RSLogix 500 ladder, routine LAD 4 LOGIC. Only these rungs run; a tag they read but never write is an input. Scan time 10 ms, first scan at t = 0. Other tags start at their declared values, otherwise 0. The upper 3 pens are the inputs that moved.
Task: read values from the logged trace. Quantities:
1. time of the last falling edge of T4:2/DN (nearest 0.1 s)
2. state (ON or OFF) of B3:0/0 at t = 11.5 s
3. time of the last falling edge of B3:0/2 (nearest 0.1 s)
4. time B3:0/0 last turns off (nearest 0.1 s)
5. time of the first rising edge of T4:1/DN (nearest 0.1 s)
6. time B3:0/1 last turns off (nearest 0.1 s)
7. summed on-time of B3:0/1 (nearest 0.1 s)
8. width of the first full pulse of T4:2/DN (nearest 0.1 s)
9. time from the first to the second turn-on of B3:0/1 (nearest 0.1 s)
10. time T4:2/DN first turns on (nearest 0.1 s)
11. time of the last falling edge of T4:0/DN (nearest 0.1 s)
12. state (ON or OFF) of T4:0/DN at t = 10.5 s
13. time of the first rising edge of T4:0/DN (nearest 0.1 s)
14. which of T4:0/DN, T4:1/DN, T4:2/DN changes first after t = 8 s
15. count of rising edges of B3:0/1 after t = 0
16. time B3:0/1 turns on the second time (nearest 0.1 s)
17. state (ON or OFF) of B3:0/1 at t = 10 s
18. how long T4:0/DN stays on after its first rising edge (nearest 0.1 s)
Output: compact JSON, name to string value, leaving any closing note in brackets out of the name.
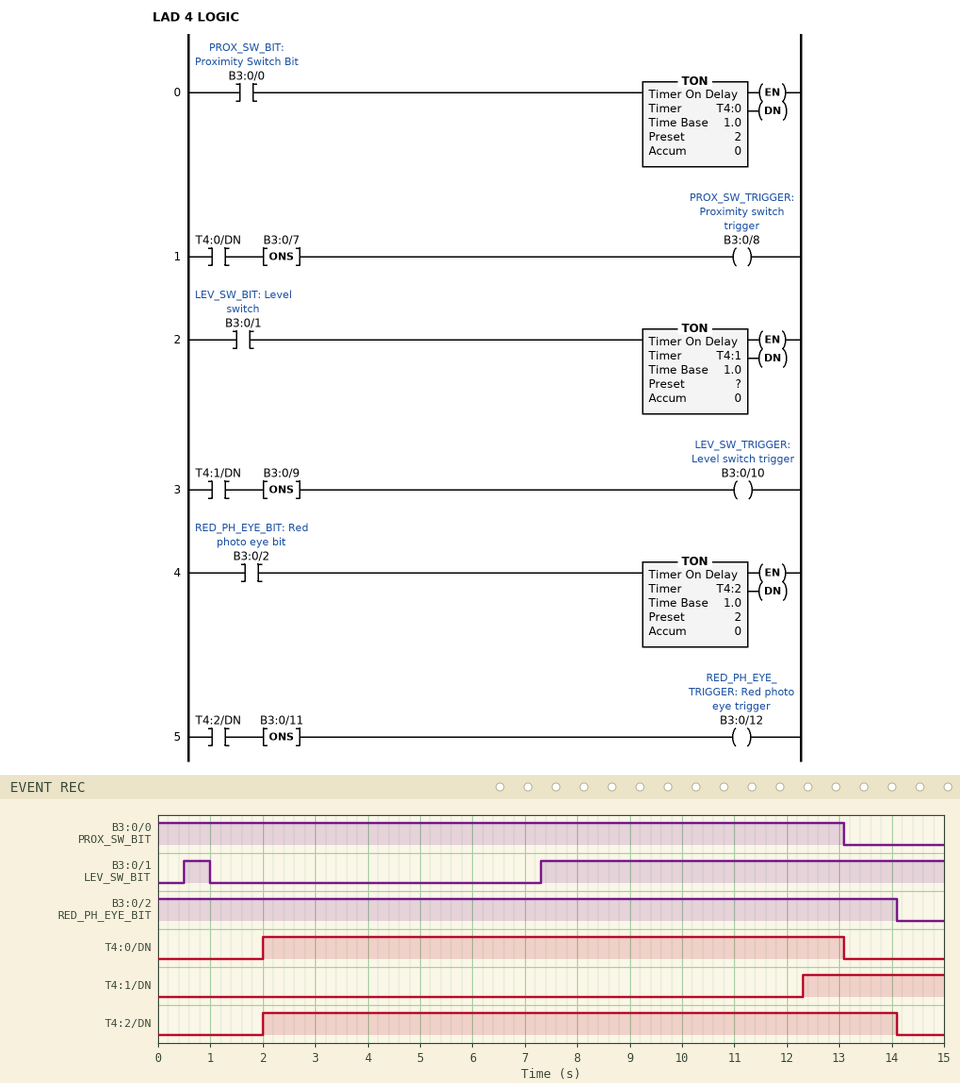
{"time of the last falling edge of T4:2/DN": "14.1 s", "state (ON or OFF) of B3:0/0 at t = 11.5 s": "ON", "time of the last falling edge of B3:0/2": "14.1 s", "time B3:0/0 last turns off": "13.1 s", "time of the first rising edge of T4:1/DN": "12.3 s", "time B3:0/1 last turns off": "1.0 s", "summed on-time of B3:0/1": "8.2 s", "width of the first full pulse of T4:2/DN": "12.1 s", "time from the first to the second turn-on of B3:0/1": "6.8 s", "time T4:2/DN first turns on": "2.0 s", "time of the last falling edge of T4:0/DN": "13.1 s", "state (ON or OFF) of T4:0/DN at t = 10.5 s": "ON", "time of the first rising edge of T4:0/DN": "2.0 s", "which of T4:0/DN, T4:1/DN, T4:2/DN changes first after t = 8 s": "T4:1/DN", "count of rising edges of B3:0/1 after t = 0": "2", "time B3:0/1 turns on the second time": "7.3 s", "state (ON or OFF) of B3:0/1 at t = 10 s": "ON", "how long T4:0/DN stays on after its first rising edge": "11.1 s"}
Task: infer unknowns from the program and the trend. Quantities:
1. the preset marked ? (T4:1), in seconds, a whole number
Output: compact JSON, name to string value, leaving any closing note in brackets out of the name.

{"the preset marked ? (T4:1), in seconds, a whole number": "5 s"}
